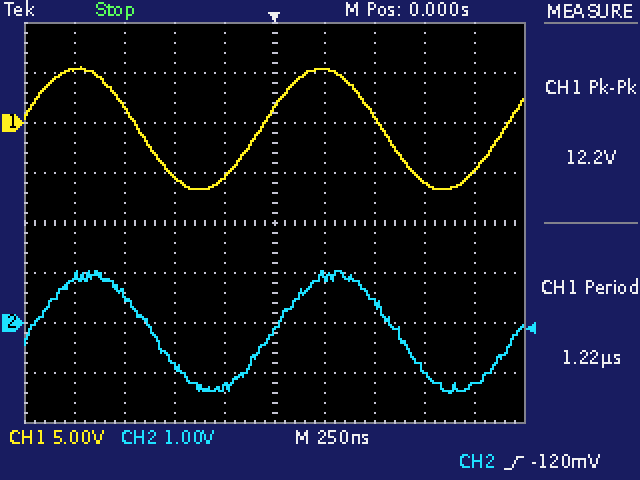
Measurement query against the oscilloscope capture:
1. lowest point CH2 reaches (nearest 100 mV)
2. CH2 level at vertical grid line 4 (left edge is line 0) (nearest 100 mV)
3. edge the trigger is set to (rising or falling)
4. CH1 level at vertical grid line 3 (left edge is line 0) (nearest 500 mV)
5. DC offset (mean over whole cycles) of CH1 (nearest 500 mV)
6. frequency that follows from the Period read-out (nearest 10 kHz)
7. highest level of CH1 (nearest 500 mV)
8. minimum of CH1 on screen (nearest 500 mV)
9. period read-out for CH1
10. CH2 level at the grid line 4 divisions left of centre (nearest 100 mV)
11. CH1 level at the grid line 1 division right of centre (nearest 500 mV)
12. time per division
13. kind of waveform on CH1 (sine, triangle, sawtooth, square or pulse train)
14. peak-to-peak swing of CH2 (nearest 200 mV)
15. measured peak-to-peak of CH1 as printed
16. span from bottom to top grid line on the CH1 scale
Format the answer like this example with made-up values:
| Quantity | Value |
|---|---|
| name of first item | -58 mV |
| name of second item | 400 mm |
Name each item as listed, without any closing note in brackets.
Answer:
| Quantity | Value |
|---|---|
| lowest point CH2 reaches | -1.4 V |
| CH2 level at vertical grid line 4 (left edge is line 0) | -1.3 V |
| edge the trigger is set to | rising |
| CH1 level at vertical grid line 3 (left edge is line 0) | -5.5 V |
| DC offset (mean over whole cycles) of CH1 | -500 mV |
| frequency that follows from the Period read-out | 820 kHz |
| highest level of CH1 | 5.5 V |
| minimum of CH1 on screen | -6.5 V |
| period read-out for CH1 | 1.22 µs |
| CH2 level at the grid line 4 divisions left of centre | 900 mV |
| CH1 level at the grid line 1 division right of centre | 5.5 V |
| time per division | 250 ns |
| kind of waveform on CH1 | sine |
| peak-to-peak swing of CH2 | 2.4 V |
| measured peak-to-peak of CH1 as printed | 12.2 V |
| span from bottom to top grid line on the CH1 scale | 40 V |
